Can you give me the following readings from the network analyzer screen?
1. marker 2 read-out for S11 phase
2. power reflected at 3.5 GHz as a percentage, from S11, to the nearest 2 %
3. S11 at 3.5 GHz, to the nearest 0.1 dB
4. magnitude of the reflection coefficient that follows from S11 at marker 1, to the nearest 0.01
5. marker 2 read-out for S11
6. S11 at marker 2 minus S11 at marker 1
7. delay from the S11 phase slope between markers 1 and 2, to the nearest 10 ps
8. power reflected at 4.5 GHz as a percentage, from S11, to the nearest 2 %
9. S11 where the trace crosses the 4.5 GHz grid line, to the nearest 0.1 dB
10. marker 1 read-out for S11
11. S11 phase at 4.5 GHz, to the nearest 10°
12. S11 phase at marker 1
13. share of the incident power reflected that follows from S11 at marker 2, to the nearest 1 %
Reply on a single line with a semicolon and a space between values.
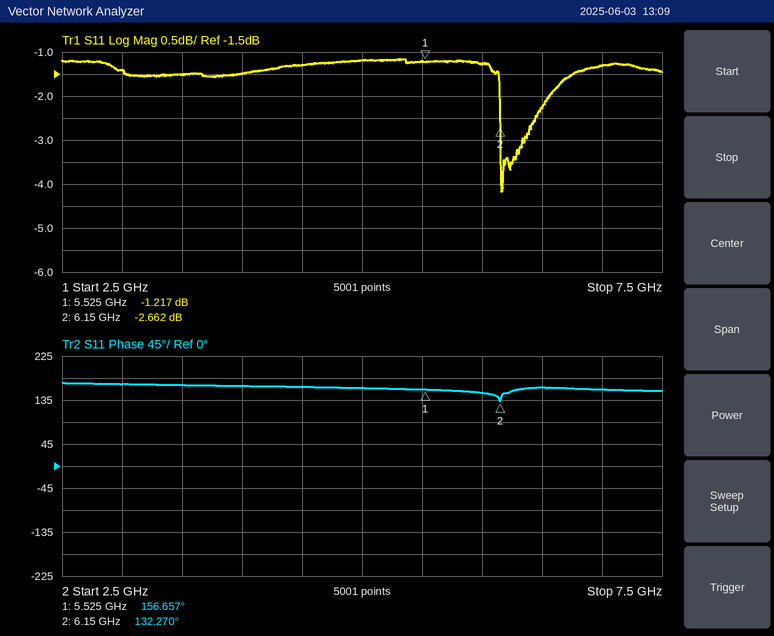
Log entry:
132.270°; 70 %; -1.5 dB; 0.87; -2.662 dB; -1.445 dB; 110 ps; 74 %; -1.3 dB; -1.217 dB; 160°; 156.657°; 54 %
